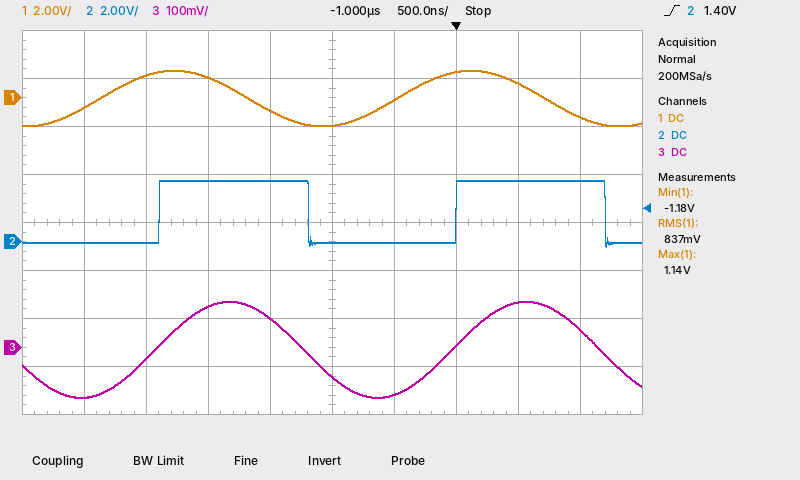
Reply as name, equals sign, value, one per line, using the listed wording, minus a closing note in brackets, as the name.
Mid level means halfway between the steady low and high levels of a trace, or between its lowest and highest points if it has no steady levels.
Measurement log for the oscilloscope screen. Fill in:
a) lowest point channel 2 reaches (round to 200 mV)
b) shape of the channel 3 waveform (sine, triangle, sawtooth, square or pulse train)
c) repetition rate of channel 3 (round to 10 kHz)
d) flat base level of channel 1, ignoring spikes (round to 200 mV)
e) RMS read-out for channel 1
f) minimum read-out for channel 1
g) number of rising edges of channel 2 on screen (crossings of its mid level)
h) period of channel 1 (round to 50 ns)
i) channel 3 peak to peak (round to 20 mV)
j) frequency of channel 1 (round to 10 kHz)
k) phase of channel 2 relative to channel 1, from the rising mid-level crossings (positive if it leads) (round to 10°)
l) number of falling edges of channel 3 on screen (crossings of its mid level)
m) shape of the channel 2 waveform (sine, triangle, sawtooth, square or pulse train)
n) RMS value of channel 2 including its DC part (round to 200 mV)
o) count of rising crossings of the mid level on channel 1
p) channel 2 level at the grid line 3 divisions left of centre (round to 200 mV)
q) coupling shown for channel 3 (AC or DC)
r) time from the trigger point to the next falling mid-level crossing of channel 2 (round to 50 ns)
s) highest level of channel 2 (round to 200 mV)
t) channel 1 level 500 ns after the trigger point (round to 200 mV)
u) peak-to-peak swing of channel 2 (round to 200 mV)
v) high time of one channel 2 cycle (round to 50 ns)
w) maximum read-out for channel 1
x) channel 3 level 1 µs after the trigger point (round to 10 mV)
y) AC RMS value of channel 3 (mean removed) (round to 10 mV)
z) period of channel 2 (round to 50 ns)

lowest point channel 2 reaches = -200 mV
shape of the channel 3 waveform = sine
repetition rate of channel 3 = 420 kHz
flat base level of channel 1, ignoring spikes = -1.2 V
RMS read-out for channel 1 = 837 mV
minimum read-out for channel 1 = -1.18 V
number of rising edges of channel 2 on screen = 2
period of channel 1 = 2.40 µs
channel 3 peak to peak = 200 mV
frequency of channel 1 = 420 kHz
phase of channel 2 relative to channel 1, from the rising mid-level crossings (positive if it leads) = -70°
number of falling edges of channel 3 on screen = 2
shape of the channel 2 waveform = square
RMS value of channel 2 including its DC part = 1.8 V
count of rising crossings of the mid level on channel 1 = 2
channel 2 level at the grid line 3 divisions left of centre = 0.0 V
coupling shown for channel 3 = DC
time from the trigger point to the next falling mid-level crossing of channel 2 = 1.20 µs
highest level of channel 2 = 2.6 V
channel 1 level 500 ns after the trigger point = 600 mV
peak-to-peak swing of channel 2 = 2.8 V
high time of one channel 2 cycle = 1.20 µs
maximum read-out for channel 1 = 1.14 V
channel 3 level 1 µs after the trigger point = 40 mV
AC RMS value of channel 3 (mean removed) = 70 mV
period of channel 2 = 2.40 µs
